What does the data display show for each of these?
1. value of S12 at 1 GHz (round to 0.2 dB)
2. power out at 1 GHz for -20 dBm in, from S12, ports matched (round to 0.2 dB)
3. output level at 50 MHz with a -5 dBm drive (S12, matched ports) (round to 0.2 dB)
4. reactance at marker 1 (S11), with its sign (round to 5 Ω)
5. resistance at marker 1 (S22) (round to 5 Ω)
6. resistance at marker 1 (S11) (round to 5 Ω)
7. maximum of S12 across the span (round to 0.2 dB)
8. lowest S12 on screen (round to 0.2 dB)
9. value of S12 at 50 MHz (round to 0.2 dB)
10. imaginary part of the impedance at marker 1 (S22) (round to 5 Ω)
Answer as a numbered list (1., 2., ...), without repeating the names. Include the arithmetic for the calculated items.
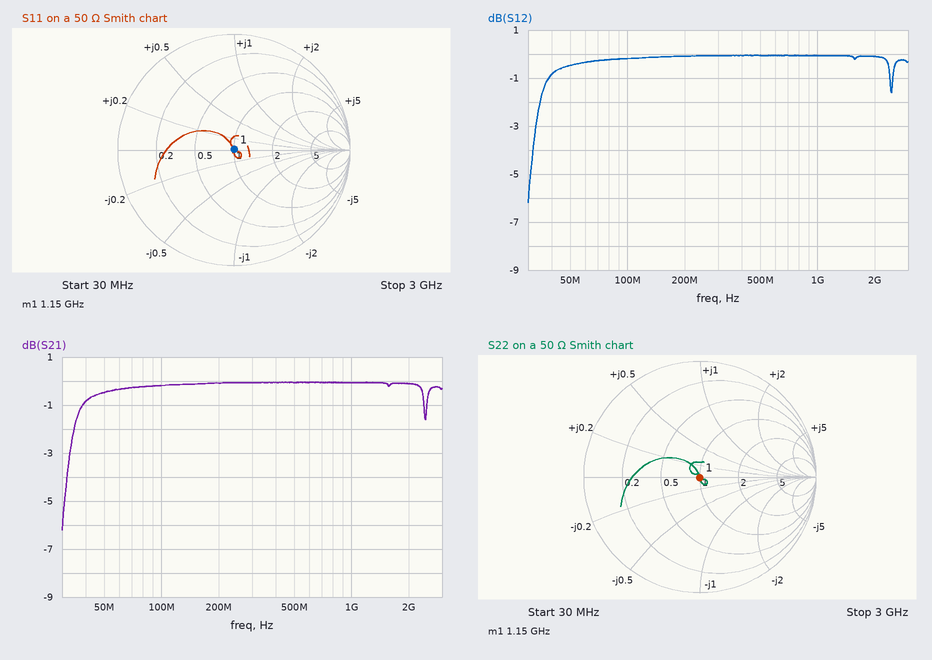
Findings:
1. 0.0 dB
2. -20 dBm + (0.0 dB) = -20.0 dBm
3. -5 dBm + (-0.4 dB) = -5.4 dBm
4. 0 Ω
5. 50 Ω
6. 50 Ω
7. 0.0 dB
8. -6.2 dB
9. -0.4 dB
10. 0 Ω
